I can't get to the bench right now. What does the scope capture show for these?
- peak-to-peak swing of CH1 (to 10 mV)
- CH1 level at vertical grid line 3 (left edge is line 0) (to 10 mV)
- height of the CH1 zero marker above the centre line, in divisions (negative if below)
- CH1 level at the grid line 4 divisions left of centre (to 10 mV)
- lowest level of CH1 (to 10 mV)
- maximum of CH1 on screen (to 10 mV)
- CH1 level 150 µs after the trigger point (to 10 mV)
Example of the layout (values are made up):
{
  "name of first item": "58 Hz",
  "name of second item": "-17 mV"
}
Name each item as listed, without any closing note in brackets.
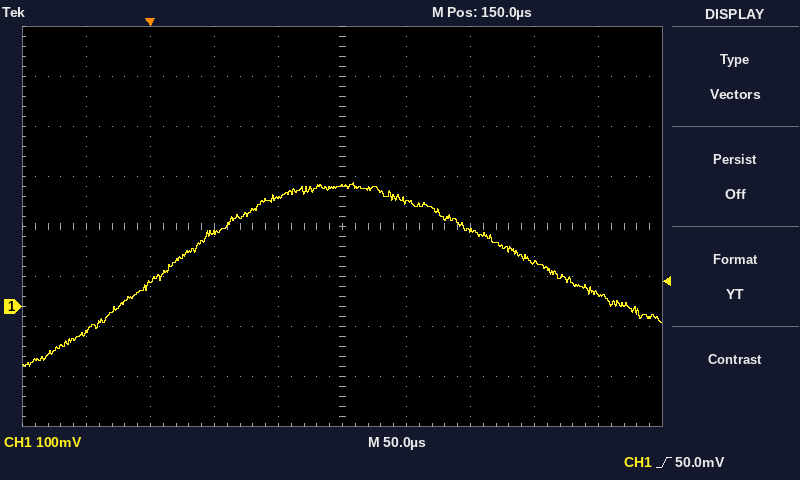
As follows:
{
  "peak-to-peak swing of CH1": "370 mV",
  "CH1 level at vertical grid line 3 (left edge is line 0)": "150 mV",
  "height of the CH1 zero marker above the centre line, in divisions": "-1.6 div",
  "CH1 level at the grid line 4 divisions left of centre": "-50 mV",
  "lowest level of CH1": "-120 mV",
  "maximum of CH1 on screen": "250 mV",
  "CH1 level 150 µs after the trigger point": "240 mV"
}
